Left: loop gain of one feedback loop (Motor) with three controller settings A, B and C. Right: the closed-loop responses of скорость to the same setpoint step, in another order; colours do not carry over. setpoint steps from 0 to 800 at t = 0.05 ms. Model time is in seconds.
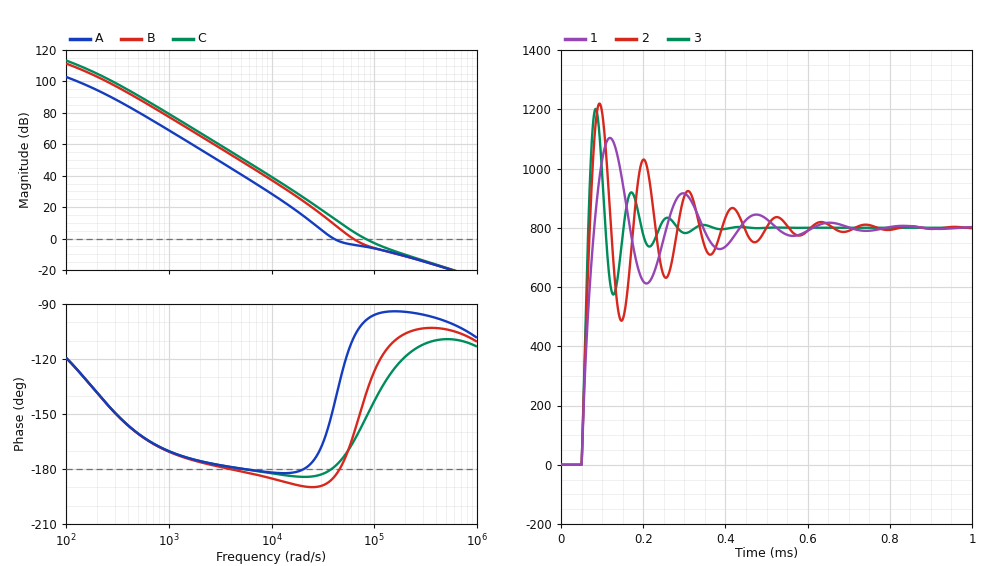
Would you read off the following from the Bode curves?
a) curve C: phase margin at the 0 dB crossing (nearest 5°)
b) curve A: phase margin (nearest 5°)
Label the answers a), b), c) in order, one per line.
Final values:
a) 25°
b) 35°
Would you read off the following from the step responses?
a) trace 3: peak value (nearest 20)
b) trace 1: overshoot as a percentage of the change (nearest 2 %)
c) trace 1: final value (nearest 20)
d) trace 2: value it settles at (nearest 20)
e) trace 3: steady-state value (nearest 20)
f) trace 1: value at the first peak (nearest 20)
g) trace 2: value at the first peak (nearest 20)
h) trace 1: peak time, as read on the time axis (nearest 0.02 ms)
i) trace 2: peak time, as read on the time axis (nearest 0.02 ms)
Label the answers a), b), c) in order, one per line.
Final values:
a) 1200
b) 38 %
c) 800
d) 800
e) 800
f) 1100
g) 1220
h) 0.12 ms
i) 0.10 ms
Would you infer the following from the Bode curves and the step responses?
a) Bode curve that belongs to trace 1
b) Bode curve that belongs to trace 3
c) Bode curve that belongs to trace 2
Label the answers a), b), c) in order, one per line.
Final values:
a) A
b) C
c) B
